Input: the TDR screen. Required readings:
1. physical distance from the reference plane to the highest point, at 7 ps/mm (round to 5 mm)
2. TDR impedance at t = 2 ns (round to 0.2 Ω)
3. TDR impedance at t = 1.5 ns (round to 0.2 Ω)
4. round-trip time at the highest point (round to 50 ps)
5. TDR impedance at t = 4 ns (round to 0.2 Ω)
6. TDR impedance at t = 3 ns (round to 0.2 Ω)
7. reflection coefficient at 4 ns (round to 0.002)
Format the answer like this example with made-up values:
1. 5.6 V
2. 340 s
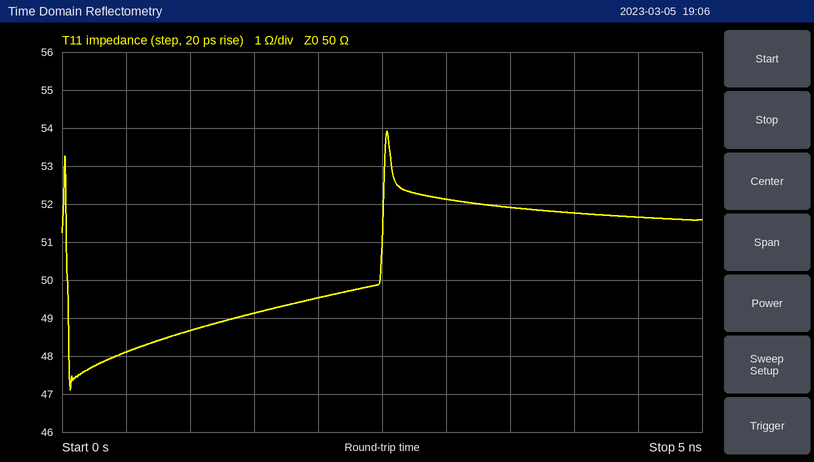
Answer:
1. 180 mm
2. 49.6 Ω
3. 49.2 Ω
4. 2.55 ns
5. 51.8 Ω
6. 52.2 Ω
7. +0.018
